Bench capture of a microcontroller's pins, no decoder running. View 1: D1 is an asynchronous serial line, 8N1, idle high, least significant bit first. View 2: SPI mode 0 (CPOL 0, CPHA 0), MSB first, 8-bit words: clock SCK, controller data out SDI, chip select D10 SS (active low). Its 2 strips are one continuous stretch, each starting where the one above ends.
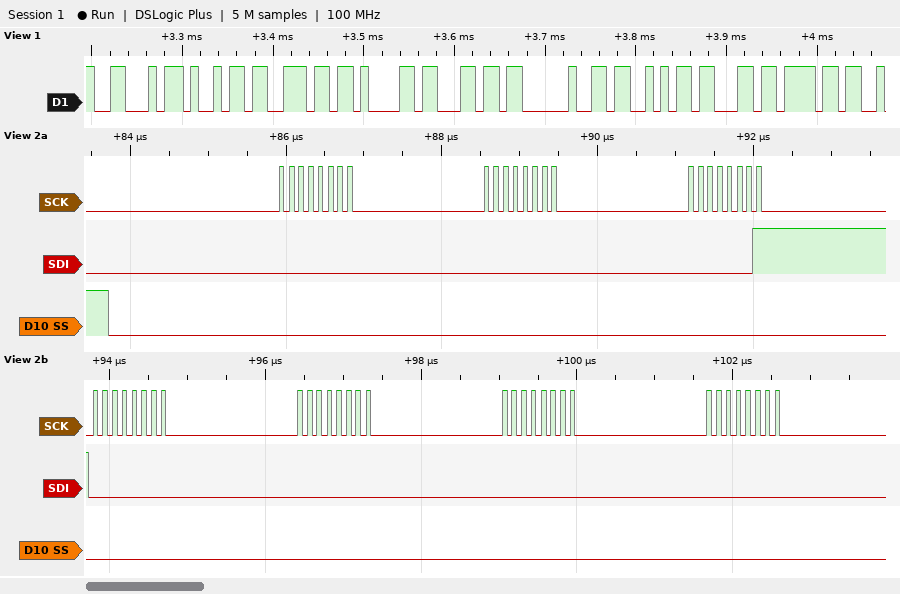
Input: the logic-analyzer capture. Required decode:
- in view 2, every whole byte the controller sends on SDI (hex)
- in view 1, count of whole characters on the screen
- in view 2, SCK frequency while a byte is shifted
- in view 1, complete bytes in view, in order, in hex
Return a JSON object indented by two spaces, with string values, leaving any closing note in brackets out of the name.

{
  "in view 2, every whole byte the controller sends on SDI": "00 00 01 00 00 00 00",
  "in view 1, count of whole characters on the screen": "9",
  "in view 2, SCK frequency while a byte is shifted": "8 MHz",
  "in view 1, complete bytes in view, in order, in hex": "46 69 6E 61 6C 20 53 63 6F"
}
